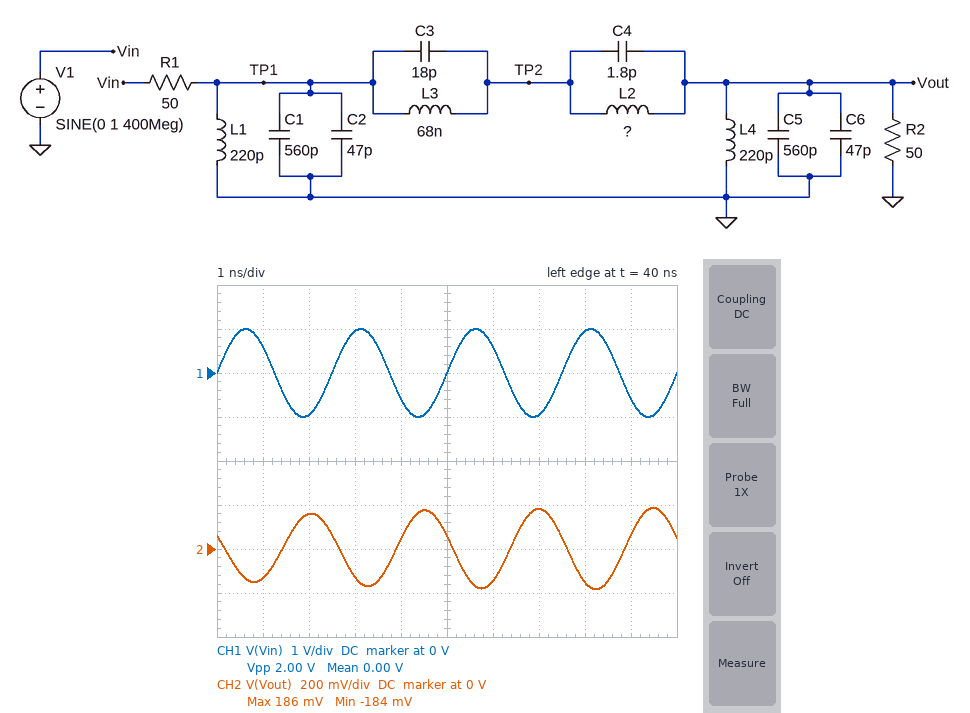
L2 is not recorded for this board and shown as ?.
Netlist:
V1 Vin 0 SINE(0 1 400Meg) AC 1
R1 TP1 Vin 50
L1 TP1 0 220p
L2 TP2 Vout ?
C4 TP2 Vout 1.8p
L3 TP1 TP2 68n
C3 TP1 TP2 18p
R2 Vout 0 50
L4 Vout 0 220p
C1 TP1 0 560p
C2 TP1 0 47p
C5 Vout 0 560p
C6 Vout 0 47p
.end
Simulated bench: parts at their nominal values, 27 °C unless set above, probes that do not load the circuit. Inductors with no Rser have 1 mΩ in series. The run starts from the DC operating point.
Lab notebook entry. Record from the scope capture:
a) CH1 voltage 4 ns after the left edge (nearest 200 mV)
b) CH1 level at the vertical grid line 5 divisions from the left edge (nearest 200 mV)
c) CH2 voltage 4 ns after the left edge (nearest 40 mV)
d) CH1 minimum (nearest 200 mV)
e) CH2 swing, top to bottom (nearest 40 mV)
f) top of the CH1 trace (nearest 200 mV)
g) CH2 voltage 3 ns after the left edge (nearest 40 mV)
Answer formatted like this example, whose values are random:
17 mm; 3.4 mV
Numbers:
-600 mV; 0 V; 40 mV; -1.0 V; 360 mV; 1.0 V; -120 mV
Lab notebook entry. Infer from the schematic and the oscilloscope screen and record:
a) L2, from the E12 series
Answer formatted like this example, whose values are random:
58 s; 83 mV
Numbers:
6.8 nH
